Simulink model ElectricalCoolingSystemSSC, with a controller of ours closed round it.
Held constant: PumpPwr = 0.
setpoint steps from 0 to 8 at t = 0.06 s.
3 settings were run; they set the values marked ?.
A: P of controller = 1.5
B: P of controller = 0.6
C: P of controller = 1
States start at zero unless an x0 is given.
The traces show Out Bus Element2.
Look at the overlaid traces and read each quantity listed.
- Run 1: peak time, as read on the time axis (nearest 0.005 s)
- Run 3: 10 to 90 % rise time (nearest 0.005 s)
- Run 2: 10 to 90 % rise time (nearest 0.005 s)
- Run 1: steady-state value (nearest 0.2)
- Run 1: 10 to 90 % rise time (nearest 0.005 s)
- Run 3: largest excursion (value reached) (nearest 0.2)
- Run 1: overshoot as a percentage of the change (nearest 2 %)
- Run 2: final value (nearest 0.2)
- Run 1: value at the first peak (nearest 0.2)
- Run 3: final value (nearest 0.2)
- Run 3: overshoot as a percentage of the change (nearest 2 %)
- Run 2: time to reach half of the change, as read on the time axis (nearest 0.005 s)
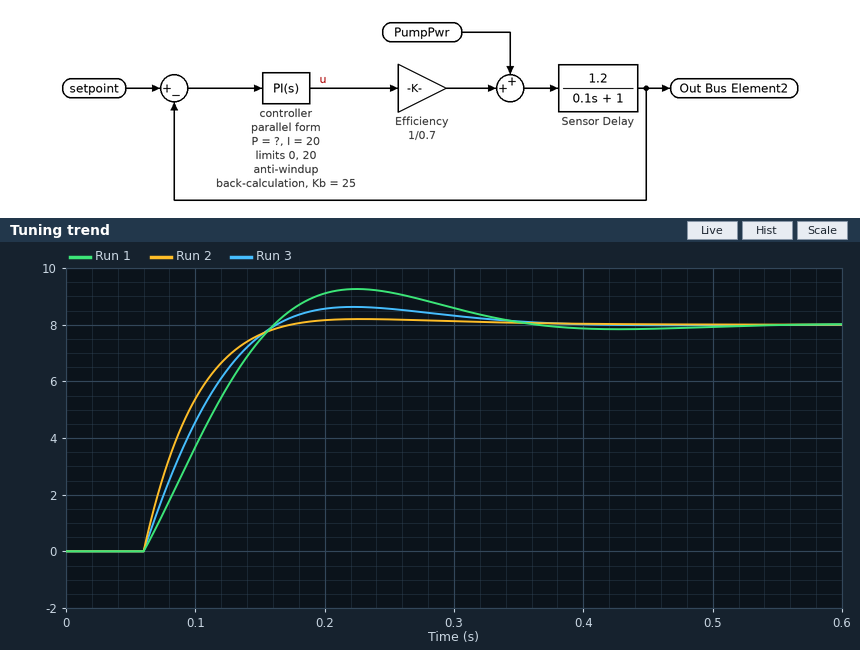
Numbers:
0.225 s
0.075 s
0.070 s
8.0
0.075 s
8.6
16 %
8.0
9.2
8.0
8 %
0.085 s
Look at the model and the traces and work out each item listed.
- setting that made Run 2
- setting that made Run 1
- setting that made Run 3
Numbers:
A
B
C
